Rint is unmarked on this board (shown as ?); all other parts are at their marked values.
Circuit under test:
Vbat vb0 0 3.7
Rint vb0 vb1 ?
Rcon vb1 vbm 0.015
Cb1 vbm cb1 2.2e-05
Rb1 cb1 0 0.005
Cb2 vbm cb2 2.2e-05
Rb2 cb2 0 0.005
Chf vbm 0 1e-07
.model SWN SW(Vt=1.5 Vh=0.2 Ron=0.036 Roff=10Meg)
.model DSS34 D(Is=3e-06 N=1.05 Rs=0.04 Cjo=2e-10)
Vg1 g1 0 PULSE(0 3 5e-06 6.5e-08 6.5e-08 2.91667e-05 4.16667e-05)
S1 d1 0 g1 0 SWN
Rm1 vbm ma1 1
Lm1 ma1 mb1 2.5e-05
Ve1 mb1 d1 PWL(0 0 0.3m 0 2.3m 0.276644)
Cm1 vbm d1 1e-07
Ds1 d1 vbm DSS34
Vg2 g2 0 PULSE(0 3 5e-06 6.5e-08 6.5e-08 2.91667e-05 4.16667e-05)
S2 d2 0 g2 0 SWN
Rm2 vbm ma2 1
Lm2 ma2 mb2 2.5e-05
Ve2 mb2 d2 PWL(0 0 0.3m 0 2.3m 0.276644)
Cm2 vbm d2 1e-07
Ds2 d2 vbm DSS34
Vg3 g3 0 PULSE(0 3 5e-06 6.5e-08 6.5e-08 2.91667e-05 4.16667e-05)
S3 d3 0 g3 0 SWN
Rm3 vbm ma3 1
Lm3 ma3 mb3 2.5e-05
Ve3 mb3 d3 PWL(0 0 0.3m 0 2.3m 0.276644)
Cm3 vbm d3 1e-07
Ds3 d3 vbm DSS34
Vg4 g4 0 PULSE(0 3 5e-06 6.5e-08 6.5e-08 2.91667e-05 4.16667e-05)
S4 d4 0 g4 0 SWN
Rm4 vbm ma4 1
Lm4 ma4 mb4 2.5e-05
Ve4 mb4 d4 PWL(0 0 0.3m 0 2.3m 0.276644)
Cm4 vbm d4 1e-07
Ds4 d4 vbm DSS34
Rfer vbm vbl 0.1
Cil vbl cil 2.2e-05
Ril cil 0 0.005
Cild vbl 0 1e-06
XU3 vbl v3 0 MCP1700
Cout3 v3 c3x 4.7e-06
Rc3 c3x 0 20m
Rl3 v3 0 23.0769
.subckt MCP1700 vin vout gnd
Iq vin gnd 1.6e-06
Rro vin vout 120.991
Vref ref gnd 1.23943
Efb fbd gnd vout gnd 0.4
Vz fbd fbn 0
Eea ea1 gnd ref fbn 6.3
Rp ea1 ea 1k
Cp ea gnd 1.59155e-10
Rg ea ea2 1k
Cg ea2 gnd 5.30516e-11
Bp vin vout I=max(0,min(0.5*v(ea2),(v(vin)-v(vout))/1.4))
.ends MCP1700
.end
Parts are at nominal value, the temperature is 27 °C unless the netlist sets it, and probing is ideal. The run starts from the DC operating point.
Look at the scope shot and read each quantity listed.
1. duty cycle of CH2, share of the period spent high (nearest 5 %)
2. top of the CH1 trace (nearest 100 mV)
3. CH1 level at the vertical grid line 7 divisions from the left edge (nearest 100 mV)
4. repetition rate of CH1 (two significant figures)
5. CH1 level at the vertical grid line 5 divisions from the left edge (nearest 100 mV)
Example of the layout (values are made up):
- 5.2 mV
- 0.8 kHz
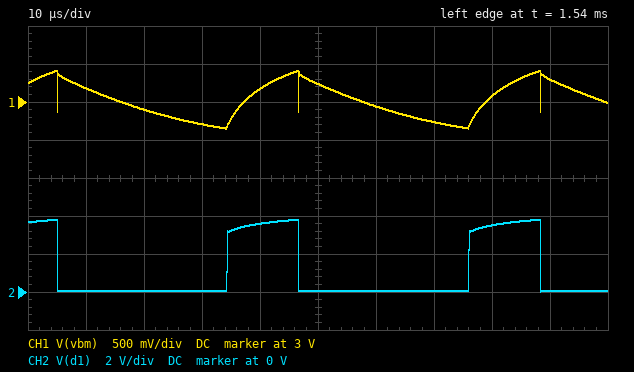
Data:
- 30 %
- 3.4 V
- 2.7 V
- 24 kHz
- 3.2 V
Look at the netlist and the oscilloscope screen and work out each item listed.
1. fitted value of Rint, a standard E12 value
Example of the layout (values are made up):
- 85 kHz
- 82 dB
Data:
- 0.12 Ω
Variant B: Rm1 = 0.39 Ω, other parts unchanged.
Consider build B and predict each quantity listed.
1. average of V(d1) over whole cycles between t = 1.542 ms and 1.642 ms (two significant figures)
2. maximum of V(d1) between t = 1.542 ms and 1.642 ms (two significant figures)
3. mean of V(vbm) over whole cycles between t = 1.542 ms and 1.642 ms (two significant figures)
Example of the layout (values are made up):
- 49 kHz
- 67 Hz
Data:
- 1.2 V
- 3.9 V
- 2.8 V
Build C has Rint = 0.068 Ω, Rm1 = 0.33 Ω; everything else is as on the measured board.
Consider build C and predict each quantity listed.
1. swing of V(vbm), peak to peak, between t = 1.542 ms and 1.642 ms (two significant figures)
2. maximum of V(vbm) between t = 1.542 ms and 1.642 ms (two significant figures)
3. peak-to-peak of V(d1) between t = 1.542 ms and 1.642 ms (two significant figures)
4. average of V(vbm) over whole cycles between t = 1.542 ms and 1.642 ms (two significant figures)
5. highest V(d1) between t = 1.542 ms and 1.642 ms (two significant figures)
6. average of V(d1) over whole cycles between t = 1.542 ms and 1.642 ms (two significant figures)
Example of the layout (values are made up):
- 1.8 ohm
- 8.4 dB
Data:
- 820 mV
- 3.6 V
- 4.0 V
- 3.1 V
- 4.1 V
- 1.3 V
